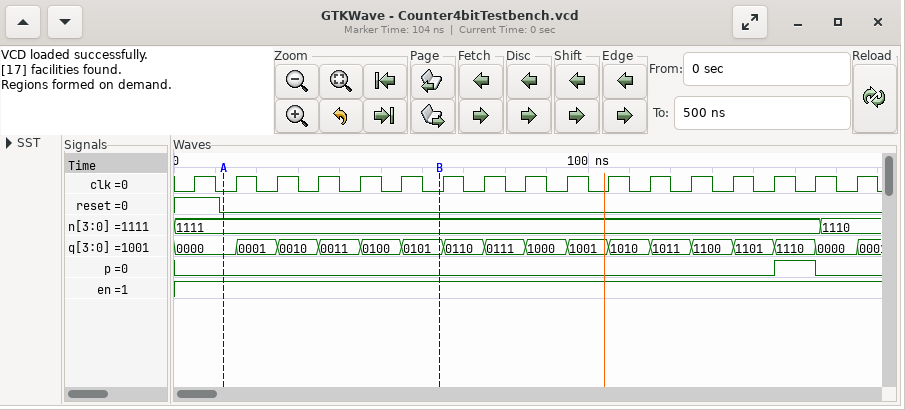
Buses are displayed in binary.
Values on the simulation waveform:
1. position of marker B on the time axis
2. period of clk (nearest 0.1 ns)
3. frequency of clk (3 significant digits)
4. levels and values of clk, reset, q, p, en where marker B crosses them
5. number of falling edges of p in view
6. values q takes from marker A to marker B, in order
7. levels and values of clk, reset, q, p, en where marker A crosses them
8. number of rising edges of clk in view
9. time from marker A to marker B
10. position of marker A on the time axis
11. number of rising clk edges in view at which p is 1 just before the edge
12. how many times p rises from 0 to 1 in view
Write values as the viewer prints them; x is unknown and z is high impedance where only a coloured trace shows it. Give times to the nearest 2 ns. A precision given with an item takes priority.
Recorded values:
64 ns
10 ns
100 MHz
clk=0, reset=0, q=0101, p=0, en=1
1
0000, 0001, 0010, 0011, 0100, 0101
clk=0, reset=0, q=0000, p=0, en=1
17
52 ns
12 ns
1
1
